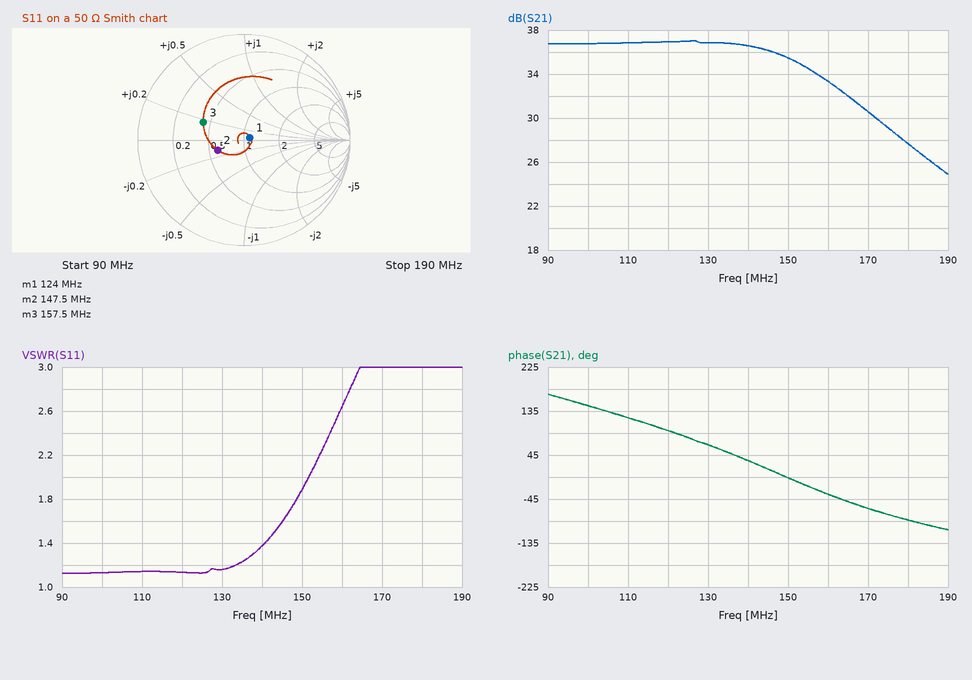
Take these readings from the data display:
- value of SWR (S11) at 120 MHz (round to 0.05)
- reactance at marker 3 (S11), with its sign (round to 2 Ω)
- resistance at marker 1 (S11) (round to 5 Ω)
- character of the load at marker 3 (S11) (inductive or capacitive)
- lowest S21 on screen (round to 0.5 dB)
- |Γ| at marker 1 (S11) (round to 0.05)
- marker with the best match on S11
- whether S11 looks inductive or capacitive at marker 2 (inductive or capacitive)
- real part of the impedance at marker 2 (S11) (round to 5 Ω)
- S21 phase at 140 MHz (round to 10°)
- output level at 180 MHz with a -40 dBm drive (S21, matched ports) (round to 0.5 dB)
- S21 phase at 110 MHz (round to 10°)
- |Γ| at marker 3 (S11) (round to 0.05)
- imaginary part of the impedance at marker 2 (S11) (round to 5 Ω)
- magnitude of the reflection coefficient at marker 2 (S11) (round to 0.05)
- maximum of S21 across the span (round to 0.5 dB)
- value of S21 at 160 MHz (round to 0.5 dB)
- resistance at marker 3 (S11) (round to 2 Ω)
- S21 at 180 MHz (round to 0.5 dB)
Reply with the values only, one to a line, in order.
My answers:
1.15
+8 Ω
55 Ω
inductive
25.0 dB
0.05
marker 1
capacitive
30 Ω
30°
-12.5 dBm
120°
0.40
-5 Ω
0.25
37.0 dB
33.5 dB
22 Ω
27.5 dB
